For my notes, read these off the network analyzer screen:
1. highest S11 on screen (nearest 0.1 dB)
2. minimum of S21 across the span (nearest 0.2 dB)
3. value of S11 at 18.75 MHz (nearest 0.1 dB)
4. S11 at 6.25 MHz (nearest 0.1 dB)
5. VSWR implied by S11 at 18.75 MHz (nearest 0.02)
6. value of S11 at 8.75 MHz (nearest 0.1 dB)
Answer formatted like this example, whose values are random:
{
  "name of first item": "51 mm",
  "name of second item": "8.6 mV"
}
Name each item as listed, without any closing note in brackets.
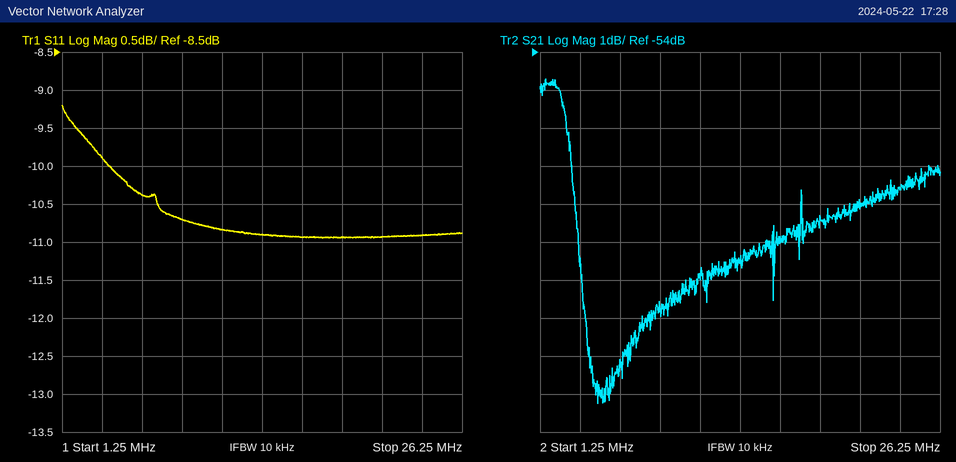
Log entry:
{
  "highest S11 on screen": "-9.2 dB",
  "minimum of S21 across the span": "-63.2 dB",
  "value of S11 at 18.75 MHz": "-10.9 dB",
  "S11 at 6.25 MHz": "-10.4 dB",
  "VSWR implied by S11 at 18.75 MHz": "1.80",
  "value of S11 at 8.75 MHz": "-10.7 dB"
}
